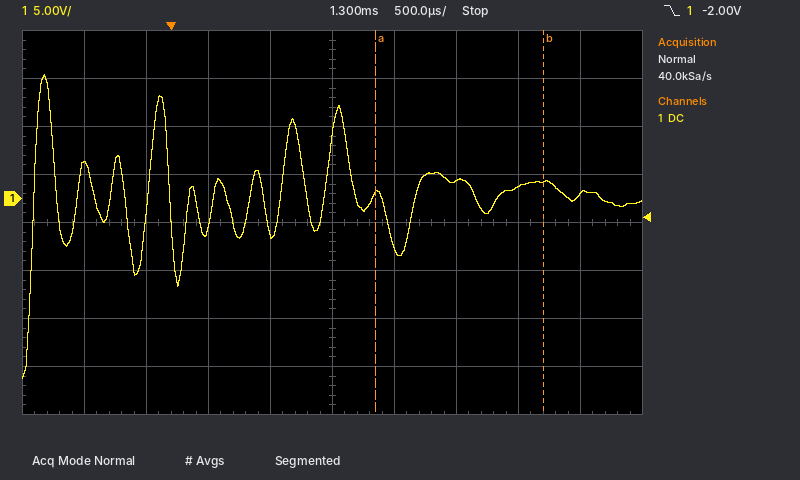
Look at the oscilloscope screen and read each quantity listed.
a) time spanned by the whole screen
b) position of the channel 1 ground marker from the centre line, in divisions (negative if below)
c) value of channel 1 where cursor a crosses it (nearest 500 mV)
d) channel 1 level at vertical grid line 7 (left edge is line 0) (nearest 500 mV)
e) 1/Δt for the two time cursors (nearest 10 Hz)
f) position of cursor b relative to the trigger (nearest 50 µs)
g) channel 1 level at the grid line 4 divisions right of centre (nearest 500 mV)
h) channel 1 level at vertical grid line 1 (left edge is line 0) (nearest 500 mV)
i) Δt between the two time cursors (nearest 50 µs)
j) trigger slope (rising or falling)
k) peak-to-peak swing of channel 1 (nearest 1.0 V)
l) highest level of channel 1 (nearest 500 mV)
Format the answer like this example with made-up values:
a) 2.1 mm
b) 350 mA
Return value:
a) 5 ms
b) +0.5 div
c) 500 mV
d) 2.0 V
e) 740 Hz
f) +3.00 ms
g) 500 mV
h) 3.5 V
i) 1.35 ms
j) falling
k) 32.0 V
l) 13.0 V
